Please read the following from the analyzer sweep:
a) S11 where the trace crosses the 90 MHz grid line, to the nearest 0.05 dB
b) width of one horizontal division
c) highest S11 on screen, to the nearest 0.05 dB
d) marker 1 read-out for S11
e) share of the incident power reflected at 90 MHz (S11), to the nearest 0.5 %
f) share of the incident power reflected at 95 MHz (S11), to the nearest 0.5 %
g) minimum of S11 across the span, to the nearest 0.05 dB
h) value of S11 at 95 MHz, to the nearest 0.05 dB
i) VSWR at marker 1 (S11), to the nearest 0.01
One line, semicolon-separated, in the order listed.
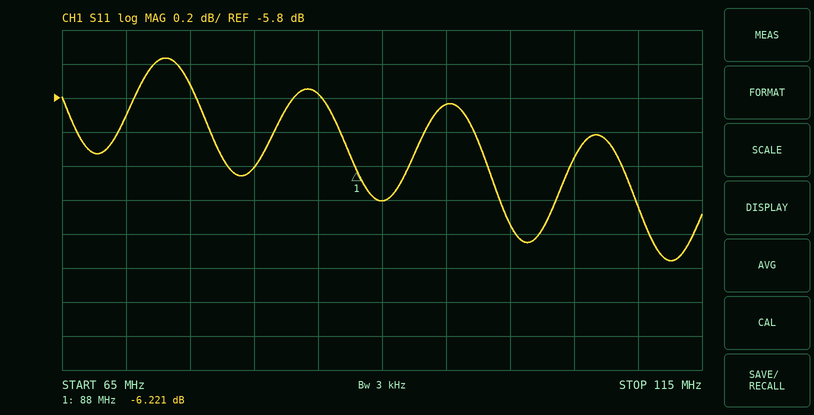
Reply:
-6.40 dB; 5 MHz; -5.55 dB; -6.221 dB; 23.0 %; 26.0 %; -6.75 dB; -5.85 dB; 2.91
